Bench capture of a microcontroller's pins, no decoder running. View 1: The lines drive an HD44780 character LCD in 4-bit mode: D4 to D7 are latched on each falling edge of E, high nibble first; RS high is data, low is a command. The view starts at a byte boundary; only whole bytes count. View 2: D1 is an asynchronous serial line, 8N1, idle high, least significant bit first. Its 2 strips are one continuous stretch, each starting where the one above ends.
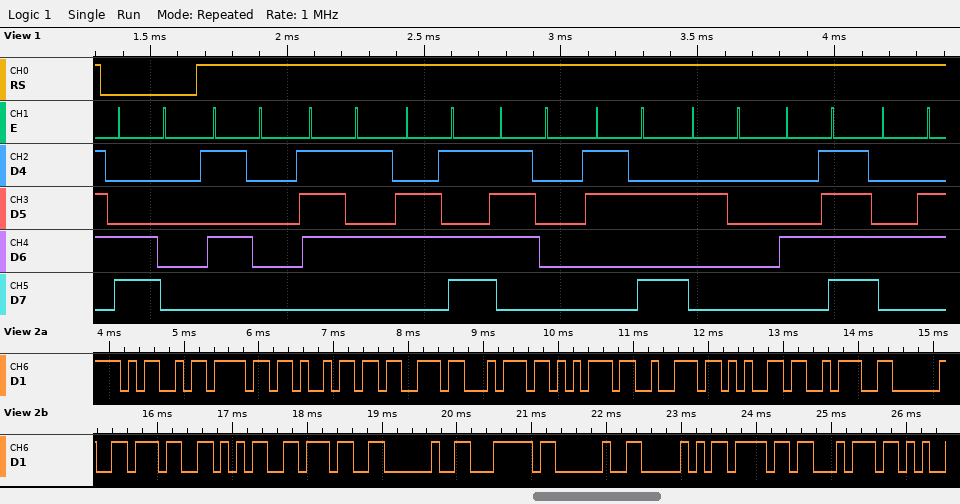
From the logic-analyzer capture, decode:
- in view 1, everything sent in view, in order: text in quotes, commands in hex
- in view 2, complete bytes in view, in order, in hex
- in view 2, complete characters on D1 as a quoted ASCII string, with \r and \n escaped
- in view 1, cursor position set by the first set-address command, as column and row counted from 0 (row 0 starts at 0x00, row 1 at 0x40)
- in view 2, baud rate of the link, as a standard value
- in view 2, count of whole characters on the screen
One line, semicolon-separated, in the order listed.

0xC0 "Pump: OF"; 4D 6F 69 73 74 75 72 65 3A 20 37 35 37 20 7C 20 50 6F 74; "Moisture: 757 | Pot"; column 0, row 1; 9600 baud; 19
